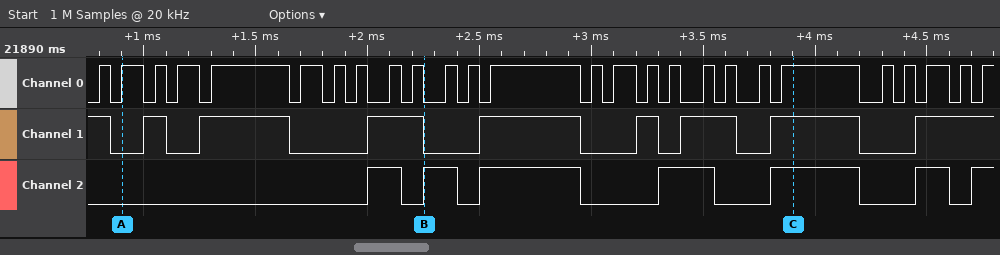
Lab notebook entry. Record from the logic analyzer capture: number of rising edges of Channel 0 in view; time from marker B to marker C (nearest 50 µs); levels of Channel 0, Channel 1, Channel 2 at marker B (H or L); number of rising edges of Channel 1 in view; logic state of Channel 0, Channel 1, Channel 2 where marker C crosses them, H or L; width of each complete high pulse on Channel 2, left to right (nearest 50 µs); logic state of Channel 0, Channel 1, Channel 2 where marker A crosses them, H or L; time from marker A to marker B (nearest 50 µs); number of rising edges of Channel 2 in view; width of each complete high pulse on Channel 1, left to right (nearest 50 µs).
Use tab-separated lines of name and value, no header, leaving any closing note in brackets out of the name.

number of rising edges of Channel 0 in view	26
time from marker B to marker C	1650 µs
levels of Channel 0, Channel 1, Channel 2 at marker B	Channel 0=L, Channel 1=L, Channel 2=H
number of rising edges of Channel 1 in view	8
logic state of Channel 0, Channel 1, Channel 2 where marker C crosses them, H or L	Channel 0=H, Channel 1=H, Channel 2=H
width of each complete high pulse on Channel 2, left to right	150 µs, 150 µs, 450 µs, 250 µs, 400 µs, 150 µs
logic state of Channel 0, Channel 1, Channel 2 where marker A crosses them, H or L	Channel 0=H, Channel 1=L, Channel 2=L
time from marker A to marker B	1350 µs
number of rising edges of Channel 2 in view	7
width of each complete high pulse on Channel 1, left to right	100 µs, 400 µs, 250 µs, 450 µs, 100 µs, 250 µs, 400 µs
